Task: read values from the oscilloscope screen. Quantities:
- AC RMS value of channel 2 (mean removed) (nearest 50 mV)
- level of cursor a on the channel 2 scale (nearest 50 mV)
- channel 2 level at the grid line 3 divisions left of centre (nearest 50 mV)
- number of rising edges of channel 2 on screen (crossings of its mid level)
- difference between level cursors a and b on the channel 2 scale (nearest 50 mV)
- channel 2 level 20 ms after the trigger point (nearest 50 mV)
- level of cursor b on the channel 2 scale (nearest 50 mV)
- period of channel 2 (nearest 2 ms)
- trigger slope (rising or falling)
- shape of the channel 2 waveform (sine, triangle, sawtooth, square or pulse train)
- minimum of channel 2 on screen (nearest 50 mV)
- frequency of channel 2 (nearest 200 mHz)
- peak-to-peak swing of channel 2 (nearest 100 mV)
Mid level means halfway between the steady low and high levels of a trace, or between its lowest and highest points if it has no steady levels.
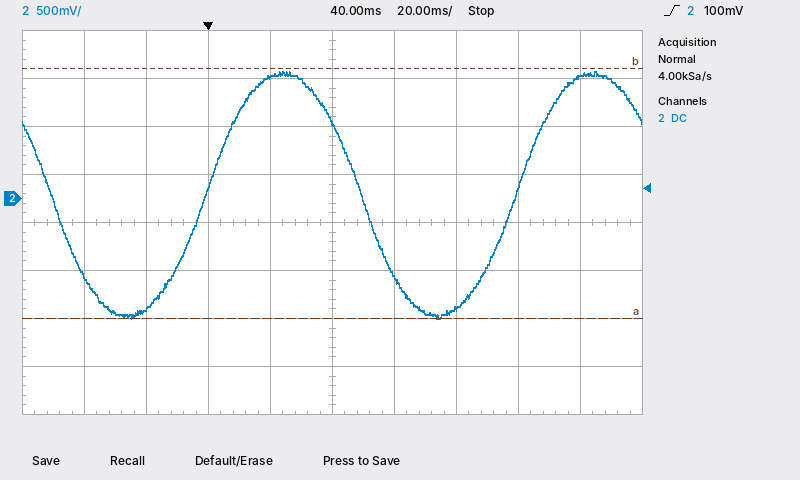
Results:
900 mV
-1.25 V
-1.15 V
2
2.60 V
1.25 V
1.35 V
100 ms
rising
sine
-1.25 V
10.0 Hz
2.60 V
